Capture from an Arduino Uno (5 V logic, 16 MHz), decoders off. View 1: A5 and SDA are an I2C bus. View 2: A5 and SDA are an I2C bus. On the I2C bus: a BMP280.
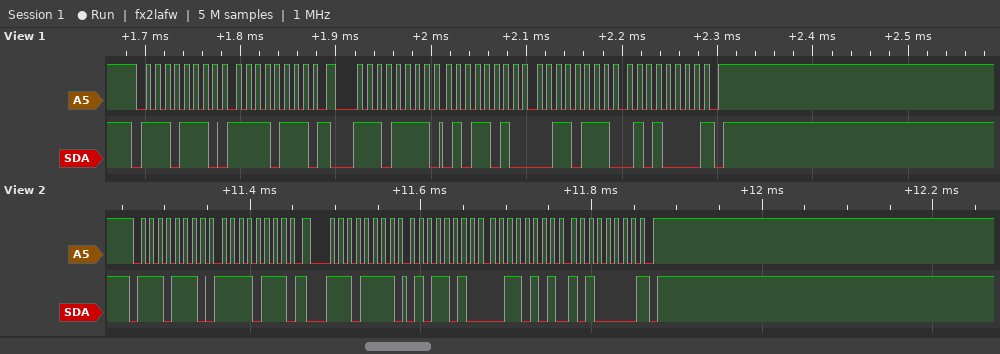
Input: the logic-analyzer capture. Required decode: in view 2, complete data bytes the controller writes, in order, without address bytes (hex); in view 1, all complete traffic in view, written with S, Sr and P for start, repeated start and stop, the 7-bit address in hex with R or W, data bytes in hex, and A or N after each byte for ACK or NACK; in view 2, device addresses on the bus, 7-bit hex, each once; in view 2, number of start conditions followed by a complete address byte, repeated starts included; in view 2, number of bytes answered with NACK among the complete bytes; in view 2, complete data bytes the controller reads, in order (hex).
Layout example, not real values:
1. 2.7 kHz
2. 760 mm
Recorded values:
1. F7
2. S 77W A F7 A Sr 77R A 5A A 37 A 50 N P
3. 0x77
4. 2
5. 1
6. 5A 35 A0
